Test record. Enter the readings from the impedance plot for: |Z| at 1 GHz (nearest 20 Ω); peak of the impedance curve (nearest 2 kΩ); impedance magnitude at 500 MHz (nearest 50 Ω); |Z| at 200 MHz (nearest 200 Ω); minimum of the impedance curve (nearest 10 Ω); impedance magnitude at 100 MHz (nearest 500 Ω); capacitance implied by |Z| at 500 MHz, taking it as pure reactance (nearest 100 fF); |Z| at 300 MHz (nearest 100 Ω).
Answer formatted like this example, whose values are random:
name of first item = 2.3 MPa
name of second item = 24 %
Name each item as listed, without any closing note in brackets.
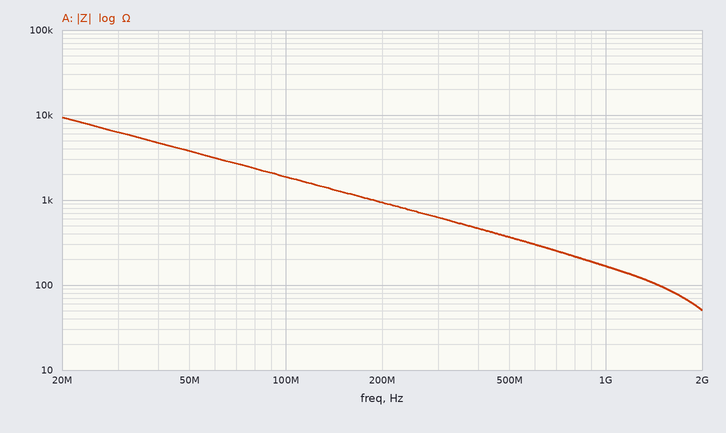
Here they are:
|Z| at 1 GHz = 160 Ω
peak of the impedance curve = 10 kΩ
impedance magnitude at 500 MHz = 350 Ω
|Z| at 200 MHz = 1.0 kΩ
minimum of the impedance curve = 50 Ω
impedance magnitude at 100 MHz = 2.0 kΩ
capacitance implied by |Z| at 500 MHz, taking it as pure reactance = 900 fF
|Z| at 300 MHz = 600 Ω
